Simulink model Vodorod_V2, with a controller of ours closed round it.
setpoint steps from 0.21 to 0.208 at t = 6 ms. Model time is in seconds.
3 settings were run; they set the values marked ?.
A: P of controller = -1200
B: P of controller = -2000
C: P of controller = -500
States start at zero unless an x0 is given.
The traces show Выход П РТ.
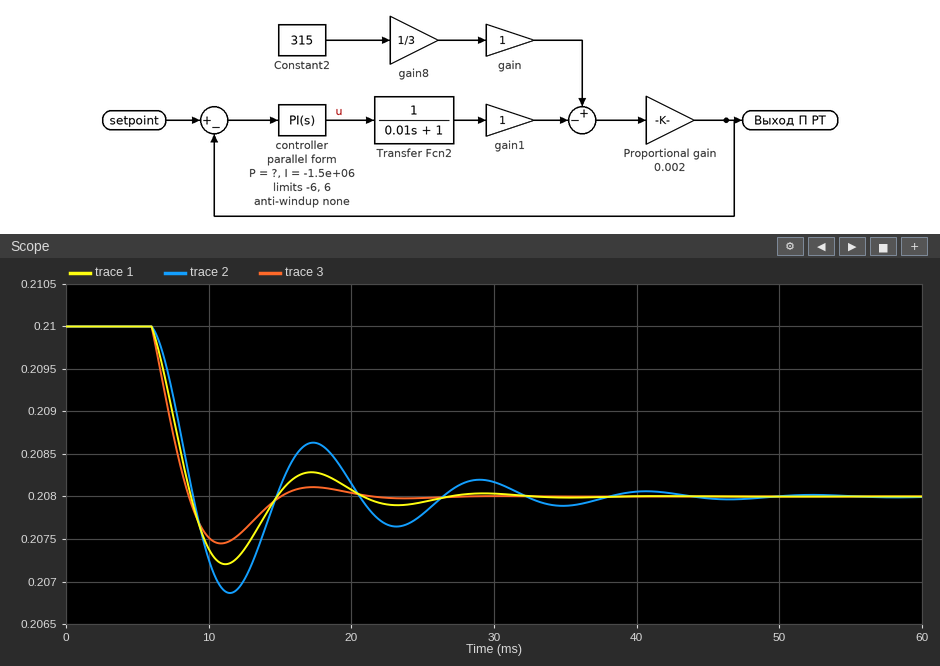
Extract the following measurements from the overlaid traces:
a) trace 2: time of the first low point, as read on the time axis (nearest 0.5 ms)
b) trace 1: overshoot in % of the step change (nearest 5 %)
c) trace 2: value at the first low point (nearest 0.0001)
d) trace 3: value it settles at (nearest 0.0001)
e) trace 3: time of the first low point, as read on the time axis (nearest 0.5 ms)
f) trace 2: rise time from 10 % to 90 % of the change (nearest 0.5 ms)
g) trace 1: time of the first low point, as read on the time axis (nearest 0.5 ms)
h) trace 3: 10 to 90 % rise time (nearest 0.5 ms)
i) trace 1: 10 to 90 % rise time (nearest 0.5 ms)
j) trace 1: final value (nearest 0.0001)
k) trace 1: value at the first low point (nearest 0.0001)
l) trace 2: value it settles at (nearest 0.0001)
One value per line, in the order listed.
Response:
11.5 ms
40 %
0.2069
0.2080
11.0 ms
2.0 ms
11.0 ms
2.0 ms
2.0 ms
0.2080
0.2072
0.2080
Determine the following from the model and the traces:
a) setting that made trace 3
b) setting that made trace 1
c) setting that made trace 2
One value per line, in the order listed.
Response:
B
A
C
